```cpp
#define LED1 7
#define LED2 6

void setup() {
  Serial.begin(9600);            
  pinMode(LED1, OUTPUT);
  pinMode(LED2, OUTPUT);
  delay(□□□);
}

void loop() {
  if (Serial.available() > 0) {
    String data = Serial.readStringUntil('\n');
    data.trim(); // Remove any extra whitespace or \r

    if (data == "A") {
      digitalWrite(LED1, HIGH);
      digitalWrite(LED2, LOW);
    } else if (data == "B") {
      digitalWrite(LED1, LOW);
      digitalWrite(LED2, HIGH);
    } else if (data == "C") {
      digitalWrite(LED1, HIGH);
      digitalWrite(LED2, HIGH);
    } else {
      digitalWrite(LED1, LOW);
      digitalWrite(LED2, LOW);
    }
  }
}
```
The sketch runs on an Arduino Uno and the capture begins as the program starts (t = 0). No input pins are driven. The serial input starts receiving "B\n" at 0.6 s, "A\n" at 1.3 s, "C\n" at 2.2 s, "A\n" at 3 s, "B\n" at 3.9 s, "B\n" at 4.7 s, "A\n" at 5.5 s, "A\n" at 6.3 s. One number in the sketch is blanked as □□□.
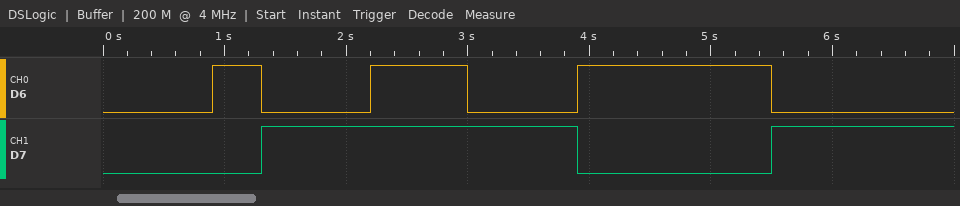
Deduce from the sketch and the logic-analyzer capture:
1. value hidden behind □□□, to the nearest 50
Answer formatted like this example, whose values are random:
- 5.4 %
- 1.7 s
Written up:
- 900
